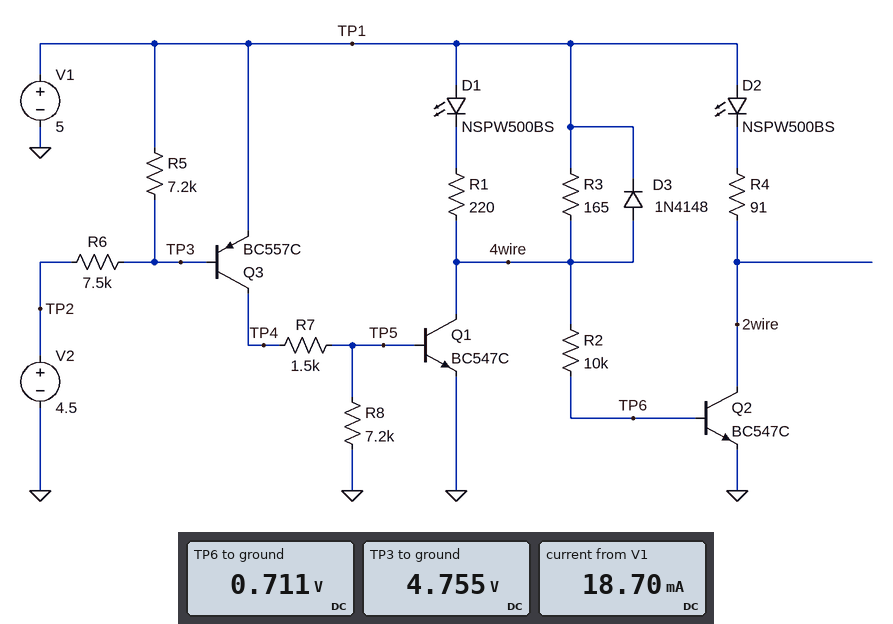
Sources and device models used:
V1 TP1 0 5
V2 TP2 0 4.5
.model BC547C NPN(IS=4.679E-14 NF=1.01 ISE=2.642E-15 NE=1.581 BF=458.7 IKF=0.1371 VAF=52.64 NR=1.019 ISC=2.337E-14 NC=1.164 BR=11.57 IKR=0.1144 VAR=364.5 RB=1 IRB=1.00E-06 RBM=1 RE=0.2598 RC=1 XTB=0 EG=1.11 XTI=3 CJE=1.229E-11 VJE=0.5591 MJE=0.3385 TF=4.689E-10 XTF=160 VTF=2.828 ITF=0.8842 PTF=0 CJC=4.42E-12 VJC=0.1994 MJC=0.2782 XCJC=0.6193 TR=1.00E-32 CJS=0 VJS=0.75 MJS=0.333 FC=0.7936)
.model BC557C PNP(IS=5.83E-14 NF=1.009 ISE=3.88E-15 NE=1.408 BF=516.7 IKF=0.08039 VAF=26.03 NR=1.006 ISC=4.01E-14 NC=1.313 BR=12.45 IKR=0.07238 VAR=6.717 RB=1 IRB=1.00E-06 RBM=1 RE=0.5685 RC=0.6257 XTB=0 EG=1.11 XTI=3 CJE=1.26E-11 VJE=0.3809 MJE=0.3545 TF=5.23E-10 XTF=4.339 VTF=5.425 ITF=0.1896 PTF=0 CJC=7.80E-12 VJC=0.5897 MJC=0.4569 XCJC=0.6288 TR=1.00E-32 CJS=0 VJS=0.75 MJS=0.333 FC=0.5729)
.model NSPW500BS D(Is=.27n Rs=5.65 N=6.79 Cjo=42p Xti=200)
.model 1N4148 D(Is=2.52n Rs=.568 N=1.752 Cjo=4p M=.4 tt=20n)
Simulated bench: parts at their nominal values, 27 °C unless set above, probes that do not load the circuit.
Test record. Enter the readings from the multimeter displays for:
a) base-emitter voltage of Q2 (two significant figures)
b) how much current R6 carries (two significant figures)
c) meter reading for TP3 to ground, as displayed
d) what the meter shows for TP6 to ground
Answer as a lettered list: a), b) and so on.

a) 710 mV
b) 34 µA
c) 4.755 V
d) 0.711 V
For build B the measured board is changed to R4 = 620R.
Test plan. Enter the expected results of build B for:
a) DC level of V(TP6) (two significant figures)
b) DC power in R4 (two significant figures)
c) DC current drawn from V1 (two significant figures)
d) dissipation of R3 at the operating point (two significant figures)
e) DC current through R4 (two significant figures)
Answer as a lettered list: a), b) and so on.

a) 680 mV
b) 7.1 mW
c) 3.8 mA
d) 30 µW
e) 3.4 mA
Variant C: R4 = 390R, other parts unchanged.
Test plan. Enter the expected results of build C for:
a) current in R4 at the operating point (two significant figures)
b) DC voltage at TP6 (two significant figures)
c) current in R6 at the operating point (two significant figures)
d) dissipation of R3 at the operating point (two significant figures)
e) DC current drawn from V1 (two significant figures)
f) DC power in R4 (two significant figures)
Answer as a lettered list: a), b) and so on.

a) 5.1 mA
b) 680 mV
c) 34 µA
d) 30 µW
e) 5.6 mA
f) 10 mW
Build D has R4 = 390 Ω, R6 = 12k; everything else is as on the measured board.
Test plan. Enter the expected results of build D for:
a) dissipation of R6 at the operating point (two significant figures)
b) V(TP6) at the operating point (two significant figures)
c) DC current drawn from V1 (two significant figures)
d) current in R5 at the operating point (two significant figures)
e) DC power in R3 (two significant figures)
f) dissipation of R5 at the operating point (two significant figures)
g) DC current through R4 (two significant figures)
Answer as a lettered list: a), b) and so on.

a) 8.1 µW
b) 680 mV
c) 5.6 mA
d) 26 µA
e) 30 µW
f) 4.9 µW
g) 5.1 mA
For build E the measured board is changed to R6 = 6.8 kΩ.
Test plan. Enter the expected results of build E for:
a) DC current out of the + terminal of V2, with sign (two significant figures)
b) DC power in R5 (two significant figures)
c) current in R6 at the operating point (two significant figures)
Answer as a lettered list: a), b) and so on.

a) -36 µA
b) 9.2 µW
c) 36 µA
